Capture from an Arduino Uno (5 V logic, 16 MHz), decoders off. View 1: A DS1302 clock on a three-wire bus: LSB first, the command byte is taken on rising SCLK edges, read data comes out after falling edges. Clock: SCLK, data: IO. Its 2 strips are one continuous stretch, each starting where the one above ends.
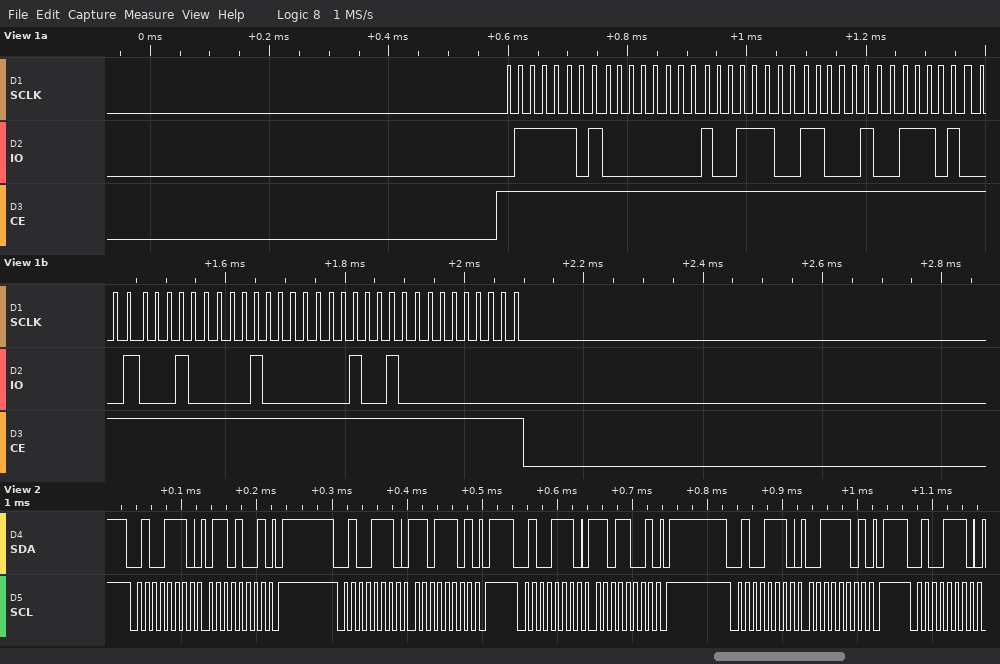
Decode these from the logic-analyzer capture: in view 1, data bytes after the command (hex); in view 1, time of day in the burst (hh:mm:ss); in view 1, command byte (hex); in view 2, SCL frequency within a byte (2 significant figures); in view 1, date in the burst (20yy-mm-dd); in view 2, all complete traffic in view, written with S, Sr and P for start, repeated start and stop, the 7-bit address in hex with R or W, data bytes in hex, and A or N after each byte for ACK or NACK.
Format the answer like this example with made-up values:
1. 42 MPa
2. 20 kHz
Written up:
1. 00 39 23 17 11 04 24 00
2. 23:39:00
3. 0xBE
4. 100 kHz
5. 2024-11-17
6. S 27W A 69 A P S 27W A DD A P S 27W A D9 A P S 27W A 3D A P S 27W A
